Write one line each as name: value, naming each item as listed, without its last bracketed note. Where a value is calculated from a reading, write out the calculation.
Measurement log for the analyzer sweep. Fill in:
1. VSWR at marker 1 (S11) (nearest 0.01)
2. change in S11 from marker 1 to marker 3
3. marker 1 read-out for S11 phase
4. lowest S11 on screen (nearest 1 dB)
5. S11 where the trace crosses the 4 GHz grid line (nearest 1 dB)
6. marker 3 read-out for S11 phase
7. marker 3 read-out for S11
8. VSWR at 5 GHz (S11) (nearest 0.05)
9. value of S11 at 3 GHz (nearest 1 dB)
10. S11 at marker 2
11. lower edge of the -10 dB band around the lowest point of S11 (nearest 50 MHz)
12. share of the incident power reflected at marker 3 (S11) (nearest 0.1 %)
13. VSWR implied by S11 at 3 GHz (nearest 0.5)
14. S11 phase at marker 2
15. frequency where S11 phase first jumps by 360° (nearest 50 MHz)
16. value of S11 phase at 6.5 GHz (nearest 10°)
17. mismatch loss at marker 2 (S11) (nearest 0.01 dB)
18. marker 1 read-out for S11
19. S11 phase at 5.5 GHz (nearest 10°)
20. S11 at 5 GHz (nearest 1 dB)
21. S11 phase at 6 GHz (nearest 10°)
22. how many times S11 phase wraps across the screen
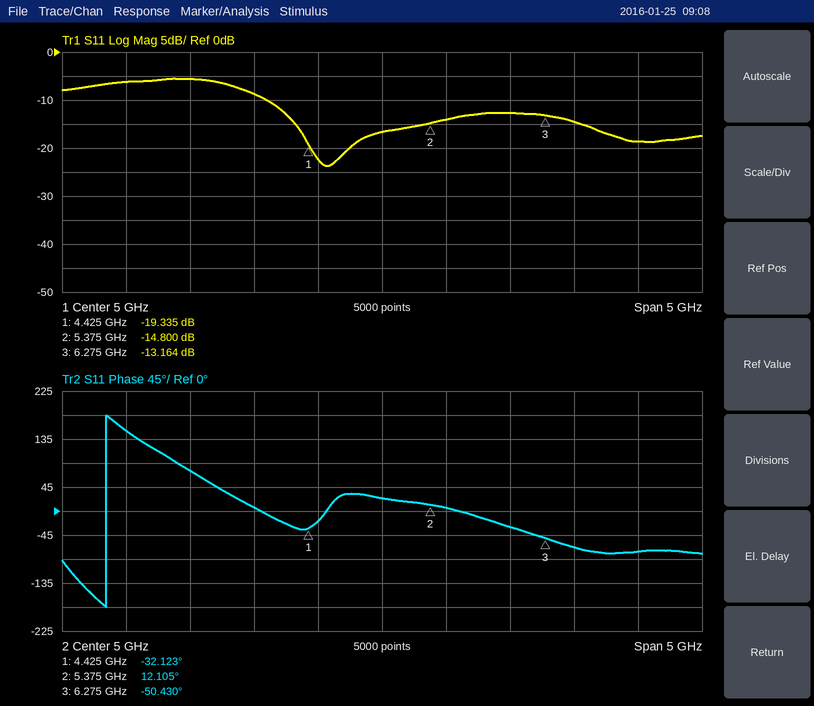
VSWR at marker 1 (S11): (1 + 0.1080)/(1 − 0.1080) ≈ 1.24
change in S11 from marker 1 to marker 3: -13.164 − (-19.335) = 6.171 dB
marker 1 read-out for S11 phase: -32.123°
lowest S11 on screen: -24 dB
S11 where the trace crosses the 4 GHz grid line: -9 dB
marker 3 read-out for S11 phase: -50.430°
marker 3 read-out for S11: -13.164 dB
VSWR at 5 GHz (S11): |Γ| = 10^(-17/20) = 0.1413; VSWR = (1 + 0.1413)/(1 − 0.1413) ≈ 1.33, so 1.35 to the nearest 0.05
value of S11 at 3 GHz: -6 dB
S11 at marker 2: -14.800 dB
lower edge of the -10 dB band around the lowest point of S11: 4.10 GHz
share of the incident power reflected at marker 3 (S11): 10^(-13.164/10) ≈ 4.8 %
VSWR implied by S11 at 3 GHz: |Γ| = 10^(-6/20) = 0.5012; VSWR = (1 + 0.5012)/(1 − 0.5012) ≈ 3.0
S11 phase at marker 2: 12.105°
frequency where S11 phase first jumps by 360°: 2.85 GHz
value of S11 phase at 6.5 GHz: -70°
mismatch loss at marker 2 (S11): −10 log10(1 − 10^(-14.8/10)) ≈ 0.15 dB
marker 1 read-out for S11: -19.335 dB
S11 phase at 5.5 GHz: 10°
S11 at 5 GHz: -17 dB
S11 phase at 6 GHz: -30°
how many times S11 phase wraps across the screen: 1
